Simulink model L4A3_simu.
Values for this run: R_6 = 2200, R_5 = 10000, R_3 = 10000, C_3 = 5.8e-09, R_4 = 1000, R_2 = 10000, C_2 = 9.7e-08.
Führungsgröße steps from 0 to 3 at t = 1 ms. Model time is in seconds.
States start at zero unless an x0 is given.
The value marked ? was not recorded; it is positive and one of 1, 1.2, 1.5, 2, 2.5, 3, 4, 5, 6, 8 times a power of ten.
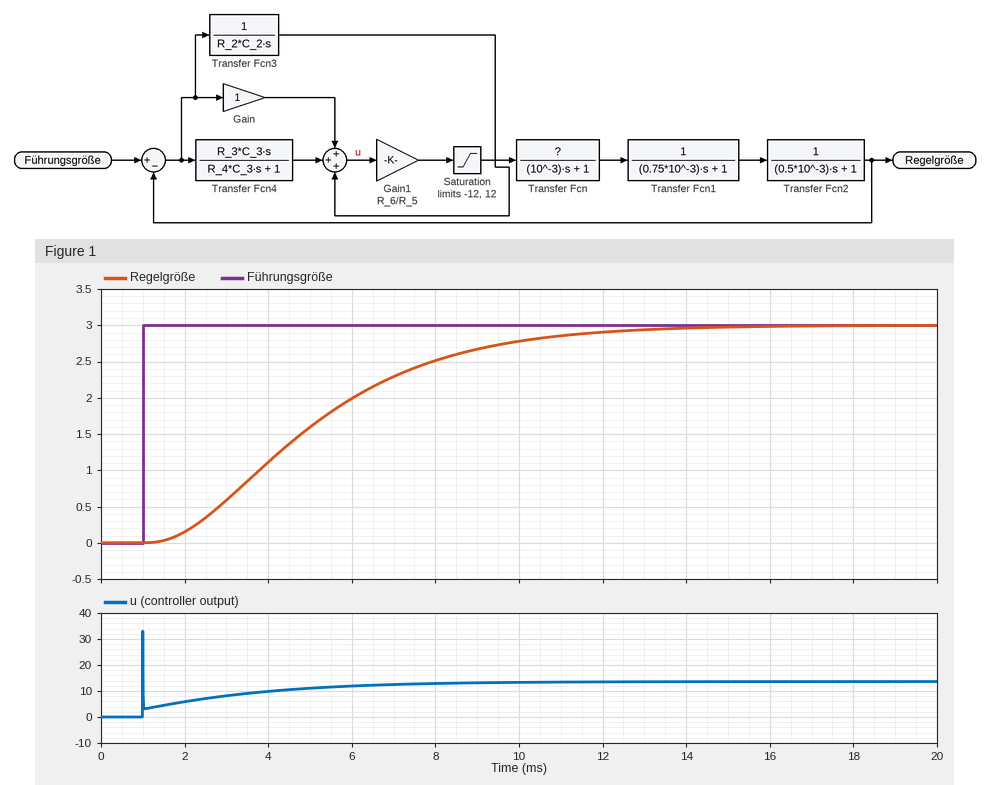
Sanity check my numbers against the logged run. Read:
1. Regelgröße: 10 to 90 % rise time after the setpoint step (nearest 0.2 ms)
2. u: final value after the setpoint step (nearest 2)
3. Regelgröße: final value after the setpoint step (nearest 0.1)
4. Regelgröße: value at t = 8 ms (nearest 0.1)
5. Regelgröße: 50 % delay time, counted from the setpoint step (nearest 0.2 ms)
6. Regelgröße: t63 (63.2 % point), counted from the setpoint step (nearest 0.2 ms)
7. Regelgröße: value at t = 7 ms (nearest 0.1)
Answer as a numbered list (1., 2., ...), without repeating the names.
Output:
1. 6.8 ms
2. 14
3. 3.0
4. 2.5
5. 3.8 ms
6. 4.8 ms
7. 2.3
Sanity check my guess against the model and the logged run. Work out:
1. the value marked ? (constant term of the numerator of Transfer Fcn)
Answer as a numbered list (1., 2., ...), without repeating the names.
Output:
1. 1
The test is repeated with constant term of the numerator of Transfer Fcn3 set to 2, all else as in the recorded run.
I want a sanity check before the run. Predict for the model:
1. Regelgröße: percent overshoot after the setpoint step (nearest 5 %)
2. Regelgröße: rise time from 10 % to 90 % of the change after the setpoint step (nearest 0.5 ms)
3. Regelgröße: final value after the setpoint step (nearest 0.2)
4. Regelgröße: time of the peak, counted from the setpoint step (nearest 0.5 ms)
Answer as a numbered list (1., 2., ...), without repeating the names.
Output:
1. 15 %
2. 3.0 ms
3. 3.0
4. 7.0 ms
